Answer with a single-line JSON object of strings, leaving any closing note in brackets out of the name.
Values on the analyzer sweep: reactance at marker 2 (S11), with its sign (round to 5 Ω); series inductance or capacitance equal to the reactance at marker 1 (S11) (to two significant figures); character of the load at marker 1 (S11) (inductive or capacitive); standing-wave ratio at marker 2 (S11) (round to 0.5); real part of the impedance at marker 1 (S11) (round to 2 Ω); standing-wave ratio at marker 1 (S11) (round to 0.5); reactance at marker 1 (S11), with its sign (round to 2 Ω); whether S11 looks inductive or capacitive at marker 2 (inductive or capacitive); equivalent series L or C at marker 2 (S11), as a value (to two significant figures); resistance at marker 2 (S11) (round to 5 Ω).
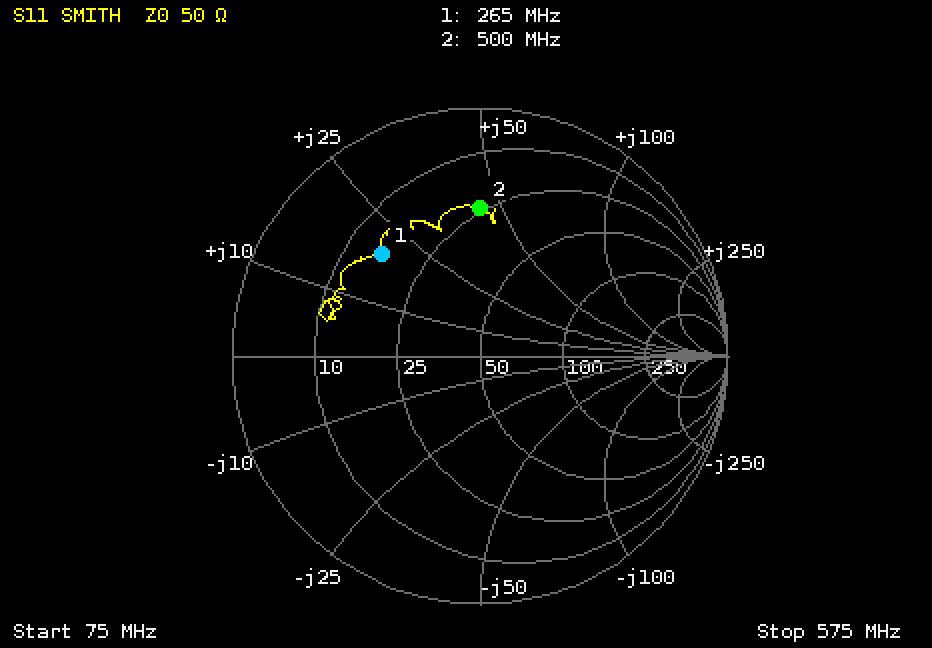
{"reactance at marker 2 (S11), with its sign": "+45 Ω", "series inductance or capacitance equal to the reactance at marker 1 (S11)": "12 nH", "character of the load at marker 1 (S11)": "inductive", "standing-wave ratio at marker 2 (S11)": "4.0", "real part of the impedance at marker 1 (S11)": "16 Ω", "standing-wave ratio at marker 1 (S11)": "3.5", "reactance at marker 1 (S11), with its sign": "+20 Ω", "whether S11 looks inductive or capacitive at marker 2": "inductive", "equivalent series L or C at marker 2 (S11), as a value": "14 nH", "resistance at marker 2 (S11)": "25 Ω"}
